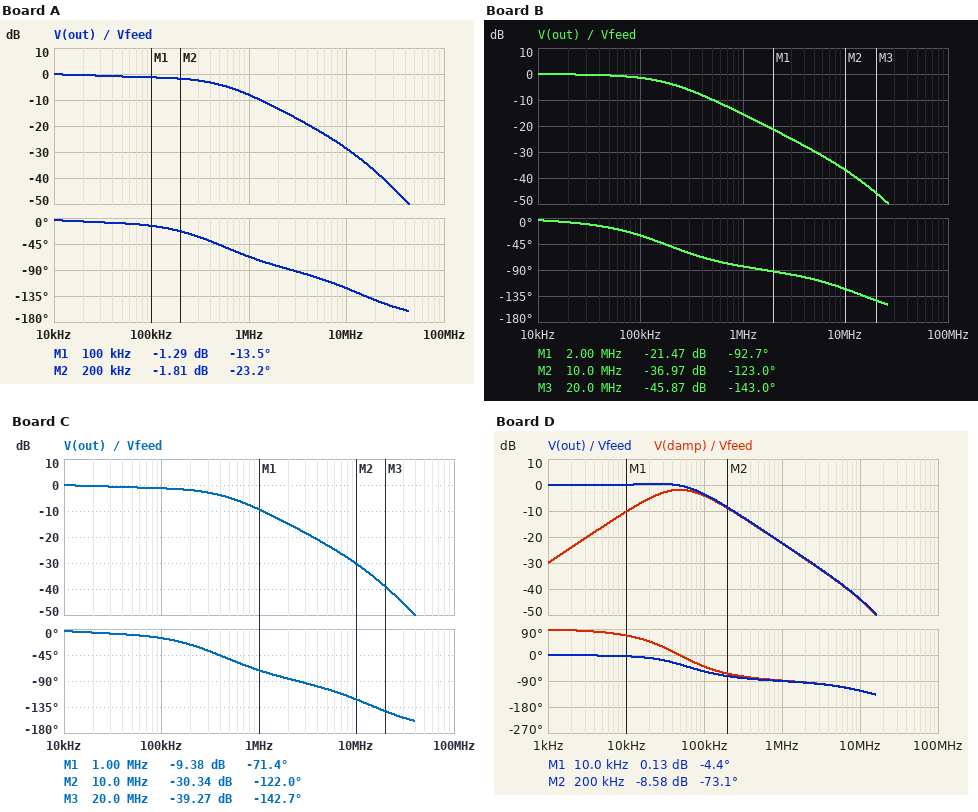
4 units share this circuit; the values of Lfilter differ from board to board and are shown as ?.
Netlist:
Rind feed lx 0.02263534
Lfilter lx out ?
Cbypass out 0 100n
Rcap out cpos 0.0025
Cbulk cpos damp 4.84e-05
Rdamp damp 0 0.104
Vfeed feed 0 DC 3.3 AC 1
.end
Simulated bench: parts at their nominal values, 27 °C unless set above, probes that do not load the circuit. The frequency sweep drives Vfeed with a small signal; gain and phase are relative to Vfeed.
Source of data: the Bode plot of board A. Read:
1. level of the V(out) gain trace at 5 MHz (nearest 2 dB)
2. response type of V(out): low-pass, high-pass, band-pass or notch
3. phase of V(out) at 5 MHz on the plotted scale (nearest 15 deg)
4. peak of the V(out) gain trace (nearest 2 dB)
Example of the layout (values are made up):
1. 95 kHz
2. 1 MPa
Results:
1. -22 dB
2. low-pass
3. -105 deg
4. 0 dB
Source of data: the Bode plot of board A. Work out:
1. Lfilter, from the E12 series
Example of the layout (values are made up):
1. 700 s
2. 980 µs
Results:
1. 39 nH
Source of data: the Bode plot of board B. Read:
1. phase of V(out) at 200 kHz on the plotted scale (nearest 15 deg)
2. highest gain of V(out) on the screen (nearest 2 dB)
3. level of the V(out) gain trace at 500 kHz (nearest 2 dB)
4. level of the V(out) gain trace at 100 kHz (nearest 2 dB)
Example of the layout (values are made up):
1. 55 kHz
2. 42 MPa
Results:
1. -45 deg
2. 0 dB
3. -10 dB
4. -2 dB
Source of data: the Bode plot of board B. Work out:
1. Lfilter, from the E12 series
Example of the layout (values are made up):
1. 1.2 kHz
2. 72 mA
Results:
1. 100 nH
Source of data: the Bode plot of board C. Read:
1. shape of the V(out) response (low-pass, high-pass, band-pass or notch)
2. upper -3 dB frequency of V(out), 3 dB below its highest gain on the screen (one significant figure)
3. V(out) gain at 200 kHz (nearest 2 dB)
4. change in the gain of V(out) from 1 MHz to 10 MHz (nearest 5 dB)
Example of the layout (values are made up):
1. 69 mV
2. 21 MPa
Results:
1. low-pass
2. 300 kHz
3. -2 dB
4. -20 dB
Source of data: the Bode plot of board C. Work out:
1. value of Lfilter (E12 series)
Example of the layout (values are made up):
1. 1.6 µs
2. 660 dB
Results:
1. 47 nH
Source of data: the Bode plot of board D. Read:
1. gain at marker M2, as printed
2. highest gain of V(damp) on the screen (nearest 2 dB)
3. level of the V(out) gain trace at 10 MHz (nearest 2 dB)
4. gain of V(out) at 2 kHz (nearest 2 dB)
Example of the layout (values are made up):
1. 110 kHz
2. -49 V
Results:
1. -8.58 dB
2. -2 dB
3. -44 dB
4. 0 dB
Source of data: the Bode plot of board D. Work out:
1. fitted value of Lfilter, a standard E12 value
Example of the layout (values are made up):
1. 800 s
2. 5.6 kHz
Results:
1. 220 nH
